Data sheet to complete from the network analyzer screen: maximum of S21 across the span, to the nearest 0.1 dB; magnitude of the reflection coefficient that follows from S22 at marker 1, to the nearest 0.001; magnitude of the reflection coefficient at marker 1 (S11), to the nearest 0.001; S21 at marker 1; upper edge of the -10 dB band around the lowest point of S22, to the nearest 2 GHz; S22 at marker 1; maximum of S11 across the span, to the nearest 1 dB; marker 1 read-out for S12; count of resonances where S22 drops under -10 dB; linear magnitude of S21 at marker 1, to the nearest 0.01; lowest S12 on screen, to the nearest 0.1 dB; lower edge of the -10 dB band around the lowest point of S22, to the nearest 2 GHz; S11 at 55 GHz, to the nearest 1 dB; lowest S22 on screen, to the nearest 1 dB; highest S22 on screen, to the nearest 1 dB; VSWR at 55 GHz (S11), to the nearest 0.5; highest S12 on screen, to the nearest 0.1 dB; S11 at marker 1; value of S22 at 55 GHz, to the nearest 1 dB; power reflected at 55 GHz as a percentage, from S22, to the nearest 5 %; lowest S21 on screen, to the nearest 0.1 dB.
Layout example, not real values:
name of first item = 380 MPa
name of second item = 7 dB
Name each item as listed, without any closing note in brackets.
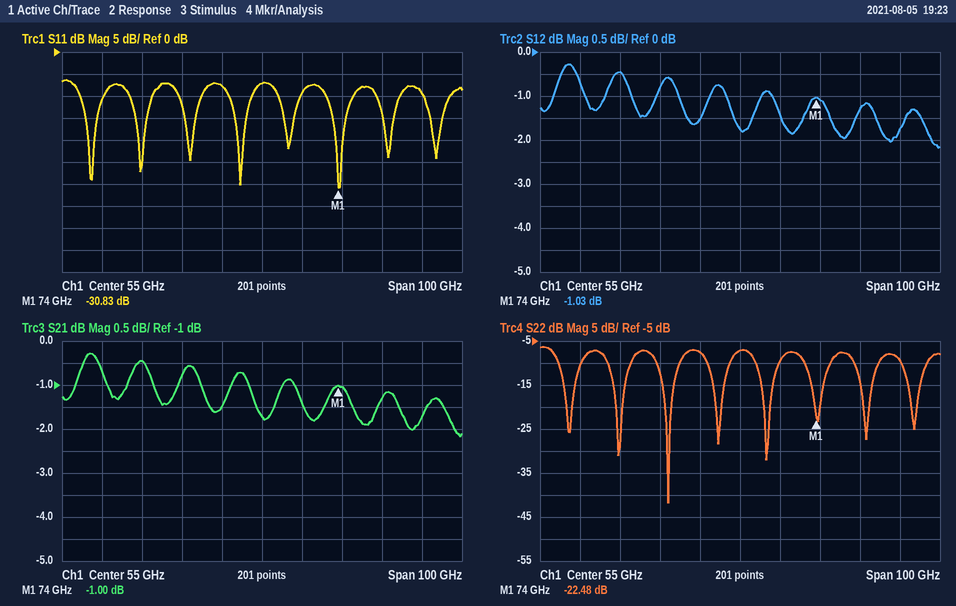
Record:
maximum of S21 across the span, to the nearest 0.1 dB = -0.3 dB
magnitude of the reflection coefficient that follows from S22 at marker 1, to the nearest 0.001 = 0.075
magnitude of the reflection coefficient at marker 1 (S11), to the nearest 0.001 = 0.029
S21 at marker 1 = -1.00 dB
upper edge of the -10 dB band around the lowest point of S22, to the nearest 2 GHz = 40 GHz
S22 at marker 1 = -22.48 dB
maximum of S11 across the span, to the nearest 1 dB = -6 dB
marker 1 read-out for S12 = -1.03 dB
count of resonances where S22 drops under -10 dB = 8
linear magnitude of S21 at marker 1, to the nearest 0.01 = 0.89
lowest S12 on screen, to the nearest 0.1 dB = -2.2 dB
lower edge of the -10 dB band around the lowest point of S22, to the nearest 2 GHz = 34 GHz
S11 at 55 GHz, to the nearest 1 dB = -7 dB
lowest S22 on screen, to the nearest 1 dB = -42 dB
highest S22 on screen, to the nearest 1 dB = -6 dB
VSWR at 55 GHz (S11), to the nearest 0.5 = 2.5
highest S12 on screen, to the nearest 0.1 dB = -0.3 dB
S11 at marker 1 = -30.83 dB
value of S22 at 55 GHz, to the nearest 1 dB = -7 dB
power reflected at 55 GHz as a percentage, from S22, to the nearest 5 % = 20 %
lowest S21 on screen, to the nearest 0.1 dB = -2.2 dB
